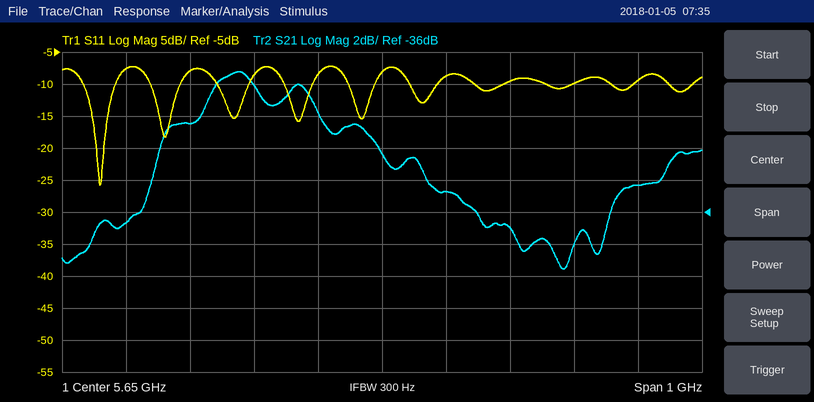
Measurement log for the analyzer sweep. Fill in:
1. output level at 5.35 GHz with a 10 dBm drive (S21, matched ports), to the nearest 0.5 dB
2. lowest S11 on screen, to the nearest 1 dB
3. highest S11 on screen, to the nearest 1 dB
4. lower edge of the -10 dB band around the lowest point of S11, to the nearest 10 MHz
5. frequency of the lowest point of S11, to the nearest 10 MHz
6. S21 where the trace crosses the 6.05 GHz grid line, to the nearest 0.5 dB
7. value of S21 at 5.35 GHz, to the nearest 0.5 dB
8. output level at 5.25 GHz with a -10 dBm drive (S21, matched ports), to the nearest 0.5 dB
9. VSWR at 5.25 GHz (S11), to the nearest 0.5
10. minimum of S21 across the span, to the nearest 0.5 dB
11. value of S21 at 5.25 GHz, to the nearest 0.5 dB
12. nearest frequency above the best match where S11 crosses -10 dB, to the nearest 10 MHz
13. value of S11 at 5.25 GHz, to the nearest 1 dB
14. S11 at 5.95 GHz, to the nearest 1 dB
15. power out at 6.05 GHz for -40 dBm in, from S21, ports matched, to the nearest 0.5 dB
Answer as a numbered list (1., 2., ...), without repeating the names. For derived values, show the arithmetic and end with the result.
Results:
1. 10 dBm + (-30.5 dB) = -20.5 dBm
2. -26 dB
3. -7 dB
4. 5.18 GHz
5. 5.21 GHz
6. -34.5 dB
7. -30.5 dB
8. -10 dBm + (-36.5 dB) = -46.5 dBm
9. |Γ| = 10^(-8/20) = 0.3981; VSWR = (1 + 0.3981)/(1 − 0.3981) ≈ 2.32, so 2.5 to the nearest 0.5
10. -39.5 dB
11. -36.5 dB
12. 5.23 GHz
13. -8 dB
14. -10 dB
15. -40 dBm + (-34.5 dB) = -74.5 dBm
